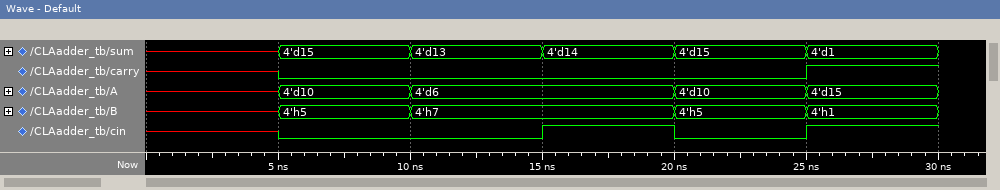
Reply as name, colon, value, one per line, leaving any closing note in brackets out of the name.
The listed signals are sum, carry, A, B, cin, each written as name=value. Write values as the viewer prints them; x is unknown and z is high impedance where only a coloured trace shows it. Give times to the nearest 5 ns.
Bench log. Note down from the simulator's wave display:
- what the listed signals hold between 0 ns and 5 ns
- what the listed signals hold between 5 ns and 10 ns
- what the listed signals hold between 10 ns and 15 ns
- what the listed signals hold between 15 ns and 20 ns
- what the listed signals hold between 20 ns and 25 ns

what the listed signals hold between 0 ns and 5 ns: sum=x, carry=x, A=x, B=x, cin=x
what the listed signals hold between 5 ns and 10 ns: sum=4'd15, carry=0, A=4'd10, B=4'h5, cin=0
what the listed signals hold between 10 ns and 15 ns: sum=4'd13, carry=0, A=4'd6, B=4'h7, cin=0
what the listed signals hold between 15 ns and 20 ns: sum=4'd14, carry=0, A=4'd6, B=4'h7, cin=1
what the listed signals hold between 20 ns and 25 ns: sum=4'd15, carry=0, A=4'd10, B=4'h5, cin=0
